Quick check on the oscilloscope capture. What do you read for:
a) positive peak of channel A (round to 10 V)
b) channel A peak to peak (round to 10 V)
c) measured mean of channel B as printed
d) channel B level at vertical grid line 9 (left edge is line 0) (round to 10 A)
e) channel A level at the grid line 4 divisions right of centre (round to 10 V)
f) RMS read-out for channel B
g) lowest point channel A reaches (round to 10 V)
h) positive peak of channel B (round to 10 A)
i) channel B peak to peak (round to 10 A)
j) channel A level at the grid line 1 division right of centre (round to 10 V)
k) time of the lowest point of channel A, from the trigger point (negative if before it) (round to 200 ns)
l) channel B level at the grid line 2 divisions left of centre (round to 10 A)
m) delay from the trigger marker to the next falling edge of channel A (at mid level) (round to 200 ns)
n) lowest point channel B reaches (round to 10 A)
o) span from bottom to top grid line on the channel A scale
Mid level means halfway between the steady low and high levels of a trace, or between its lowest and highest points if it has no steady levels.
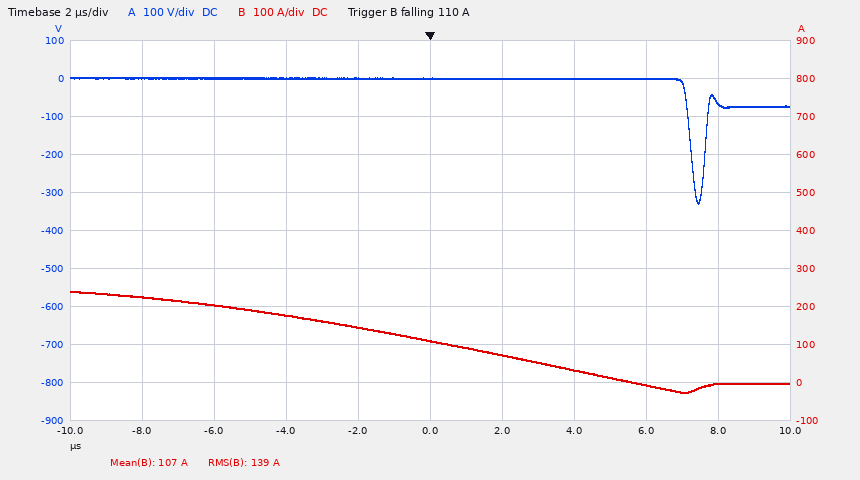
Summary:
0 V
330 V
107 A
0 A
-60 V
139 A
-330 V
240 A
270 A
0 V
+7.4 µs
180 A
7.2 µs
-30 A
1 kV
